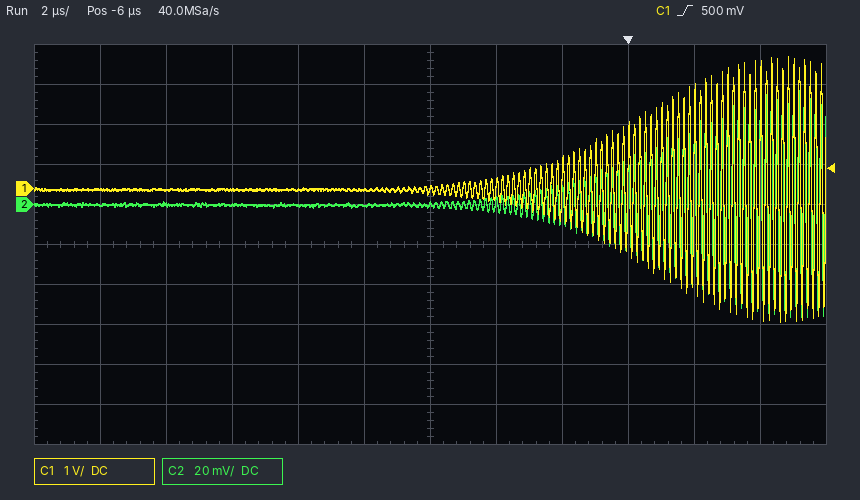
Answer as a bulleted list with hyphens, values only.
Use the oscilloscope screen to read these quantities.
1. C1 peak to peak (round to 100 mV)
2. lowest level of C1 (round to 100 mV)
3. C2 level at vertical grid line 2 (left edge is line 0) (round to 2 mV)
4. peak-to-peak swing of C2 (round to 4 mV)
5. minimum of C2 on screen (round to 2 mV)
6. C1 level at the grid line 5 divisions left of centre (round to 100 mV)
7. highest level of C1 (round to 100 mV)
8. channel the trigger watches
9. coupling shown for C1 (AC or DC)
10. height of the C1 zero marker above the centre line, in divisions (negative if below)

- 6.6 V
- -3.3 V
- 0 mV
- 112 mV
- -56 mV
- 0.0 V
- 3.3 V
- C1
- DC
- +1.4 div
